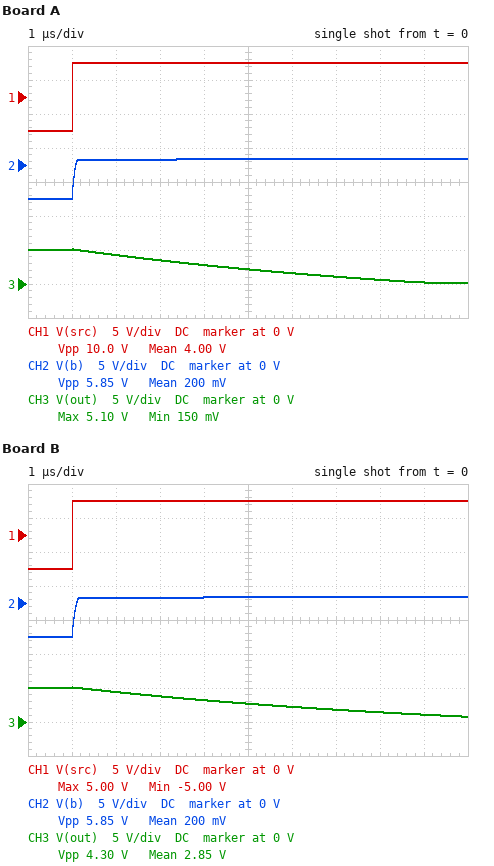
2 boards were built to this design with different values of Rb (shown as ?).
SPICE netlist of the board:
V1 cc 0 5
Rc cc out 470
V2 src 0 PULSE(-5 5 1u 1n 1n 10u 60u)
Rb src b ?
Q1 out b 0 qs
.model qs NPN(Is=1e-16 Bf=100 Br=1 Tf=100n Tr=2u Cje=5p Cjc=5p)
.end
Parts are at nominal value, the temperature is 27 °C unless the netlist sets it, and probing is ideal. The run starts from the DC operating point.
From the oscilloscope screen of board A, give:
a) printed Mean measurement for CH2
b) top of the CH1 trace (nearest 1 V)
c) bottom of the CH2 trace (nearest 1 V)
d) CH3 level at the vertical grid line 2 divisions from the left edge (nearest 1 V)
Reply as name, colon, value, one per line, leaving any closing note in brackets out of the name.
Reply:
printed Mean measurement for CH2: 200 mV
top of the CH1 trace: 5 V
bottom of the CH2 trace: -5 V
CH3 level at the vertical grid line 2 divisions from the left edge: 4 V
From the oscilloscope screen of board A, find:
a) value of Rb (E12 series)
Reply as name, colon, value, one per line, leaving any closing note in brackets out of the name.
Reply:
value of Rb: 22 kΩ
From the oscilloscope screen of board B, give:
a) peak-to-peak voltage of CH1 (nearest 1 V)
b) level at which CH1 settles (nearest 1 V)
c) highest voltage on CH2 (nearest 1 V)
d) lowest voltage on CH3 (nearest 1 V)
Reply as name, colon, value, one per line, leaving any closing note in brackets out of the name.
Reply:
peak-to-peak voltage of CH1: 10 V
level at which CH1 settles: 5 V
highest voltage on CH2: 1 V
lowest voltage on CH3: 1 V
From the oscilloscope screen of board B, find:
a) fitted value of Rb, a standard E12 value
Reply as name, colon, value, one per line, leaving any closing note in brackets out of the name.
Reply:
fitted value of Rb, a standard E12 value: 27 kΩ
